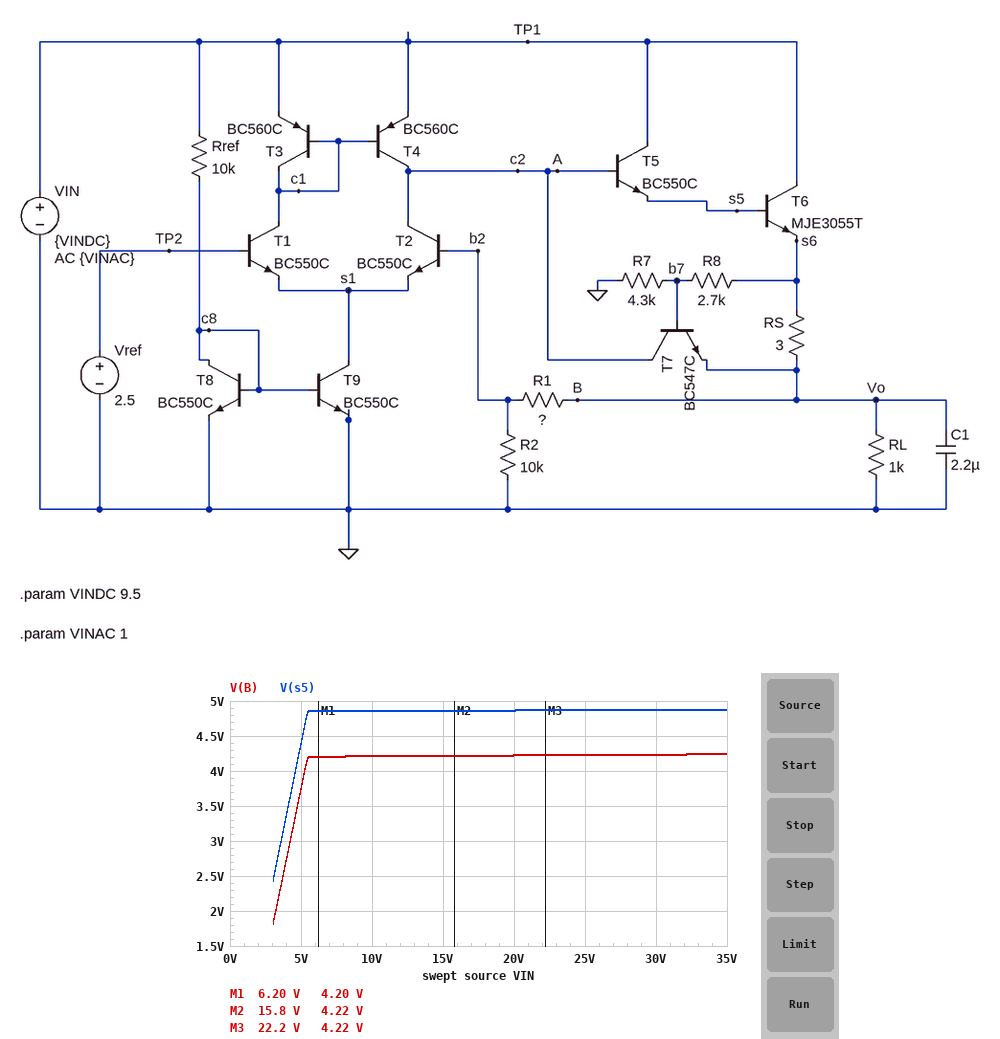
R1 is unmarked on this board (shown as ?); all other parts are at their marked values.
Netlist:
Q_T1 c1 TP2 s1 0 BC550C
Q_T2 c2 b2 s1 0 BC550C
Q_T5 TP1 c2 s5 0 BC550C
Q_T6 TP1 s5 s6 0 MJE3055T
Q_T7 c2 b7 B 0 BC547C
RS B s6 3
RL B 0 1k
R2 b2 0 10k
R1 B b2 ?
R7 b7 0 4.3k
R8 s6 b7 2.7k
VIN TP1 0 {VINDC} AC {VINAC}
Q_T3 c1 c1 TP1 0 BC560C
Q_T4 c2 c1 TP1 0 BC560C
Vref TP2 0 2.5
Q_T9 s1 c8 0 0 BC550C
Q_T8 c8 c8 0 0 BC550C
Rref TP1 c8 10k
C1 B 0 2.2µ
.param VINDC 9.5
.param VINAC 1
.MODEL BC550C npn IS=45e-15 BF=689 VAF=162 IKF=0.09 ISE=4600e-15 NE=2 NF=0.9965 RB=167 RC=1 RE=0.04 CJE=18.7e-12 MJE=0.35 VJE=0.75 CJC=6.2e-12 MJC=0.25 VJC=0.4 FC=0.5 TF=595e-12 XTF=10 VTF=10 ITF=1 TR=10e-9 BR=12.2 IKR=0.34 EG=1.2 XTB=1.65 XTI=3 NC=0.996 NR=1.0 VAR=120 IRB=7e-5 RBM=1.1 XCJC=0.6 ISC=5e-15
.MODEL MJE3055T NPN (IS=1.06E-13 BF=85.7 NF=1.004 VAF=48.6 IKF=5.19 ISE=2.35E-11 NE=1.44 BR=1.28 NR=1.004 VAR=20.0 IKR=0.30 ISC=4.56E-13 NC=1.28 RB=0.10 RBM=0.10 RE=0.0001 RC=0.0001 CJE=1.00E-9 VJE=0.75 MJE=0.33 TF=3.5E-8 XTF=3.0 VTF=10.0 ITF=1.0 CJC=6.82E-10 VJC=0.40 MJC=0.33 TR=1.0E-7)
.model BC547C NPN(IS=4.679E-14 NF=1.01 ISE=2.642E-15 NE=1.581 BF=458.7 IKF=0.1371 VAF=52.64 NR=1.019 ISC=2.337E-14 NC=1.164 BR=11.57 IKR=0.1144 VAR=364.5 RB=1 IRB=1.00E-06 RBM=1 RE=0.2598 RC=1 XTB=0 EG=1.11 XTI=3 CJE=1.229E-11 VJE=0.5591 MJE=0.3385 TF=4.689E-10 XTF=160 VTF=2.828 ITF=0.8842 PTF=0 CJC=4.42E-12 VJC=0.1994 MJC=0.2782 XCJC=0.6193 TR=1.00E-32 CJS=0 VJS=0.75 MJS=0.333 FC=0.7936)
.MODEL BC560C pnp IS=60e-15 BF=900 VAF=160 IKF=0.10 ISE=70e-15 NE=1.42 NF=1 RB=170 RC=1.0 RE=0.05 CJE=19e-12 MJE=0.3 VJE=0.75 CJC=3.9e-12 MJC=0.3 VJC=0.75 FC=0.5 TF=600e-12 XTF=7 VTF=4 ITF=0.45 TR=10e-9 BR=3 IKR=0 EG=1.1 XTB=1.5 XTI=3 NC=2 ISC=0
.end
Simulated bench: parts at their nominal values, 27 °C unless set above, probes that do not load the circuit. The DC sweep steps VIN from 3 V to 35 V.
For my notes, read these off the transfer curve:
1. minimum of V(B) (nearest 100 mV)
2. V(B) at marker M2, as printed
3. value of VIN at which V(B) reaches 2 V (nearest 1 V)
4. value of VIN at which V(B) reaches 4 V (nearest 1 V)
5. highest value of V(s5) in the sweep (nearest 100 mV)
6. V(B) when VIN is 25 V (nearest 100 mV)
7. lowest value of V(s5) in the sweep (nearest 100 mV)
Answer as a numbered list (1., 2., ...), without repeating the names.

1. 1.8 V
2. 4.22 V
3. 3 V
4. 5 V
5. 4.9 V
6. 4.2 V
7. 2.4 V
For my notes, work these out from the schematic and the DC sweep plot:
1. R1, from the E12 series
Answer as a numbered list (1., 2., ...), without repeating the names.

1. 6.8 kΩ
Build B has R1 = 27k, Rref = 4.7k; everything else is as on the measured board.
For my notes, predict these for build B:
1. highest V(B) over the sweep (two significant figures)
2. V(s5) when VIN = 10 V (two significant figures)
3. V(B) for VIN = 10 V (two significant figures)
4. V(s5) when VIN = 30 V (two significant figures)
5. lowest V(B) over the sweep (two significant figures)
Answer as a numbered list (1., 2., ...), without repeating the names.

1. 9.5 V
2. 9.4 V
3. 8.7 V
4. 10 V
5. 1.8 V
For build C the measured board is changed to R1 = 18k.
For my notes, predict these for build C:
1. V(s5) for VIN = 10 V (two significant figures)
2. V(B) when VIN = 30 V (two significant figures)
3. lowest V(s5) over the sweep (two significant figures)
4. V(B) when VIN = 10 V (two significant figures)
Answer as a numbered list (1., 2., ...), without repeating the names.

1. 7.7 V
2. 7.1 V
3. 2.4 V
4. 7.0 V
